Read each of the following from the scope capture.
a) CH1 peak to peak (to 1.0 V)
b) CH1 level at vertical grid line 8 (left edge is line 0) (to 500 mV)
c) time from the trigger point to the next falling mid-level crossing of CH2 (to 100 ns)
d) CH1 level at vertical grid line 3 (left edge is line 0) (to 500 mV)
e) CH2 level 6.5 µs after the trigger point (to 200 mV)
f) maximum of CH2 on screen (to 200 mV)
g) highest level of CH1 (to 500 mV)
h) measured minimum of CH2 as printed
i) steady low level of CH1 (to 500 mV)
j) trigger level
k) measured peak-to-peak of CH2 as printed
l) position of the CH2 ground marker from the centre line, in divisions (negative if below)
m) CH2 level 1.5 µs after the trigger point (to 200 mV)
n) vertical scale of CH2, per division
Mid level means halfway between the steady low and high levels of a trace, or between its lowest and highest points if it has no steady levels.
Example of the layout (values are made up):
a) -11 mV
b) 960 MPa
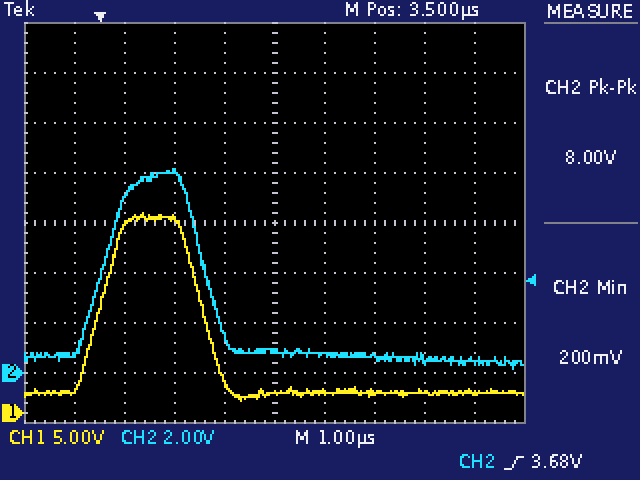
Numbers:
a) 19.0 V
b) 2.0 V
c) 2.1 µs
d) 19.5 V
e) 600 mV
f) 8.2 V
g) 20.0 V
h) 200 mV
i) 2.0 V
j) 3.68 V
k) 8.00 V
l) -3.0 div
m) 8.0 V
n) 2 V
